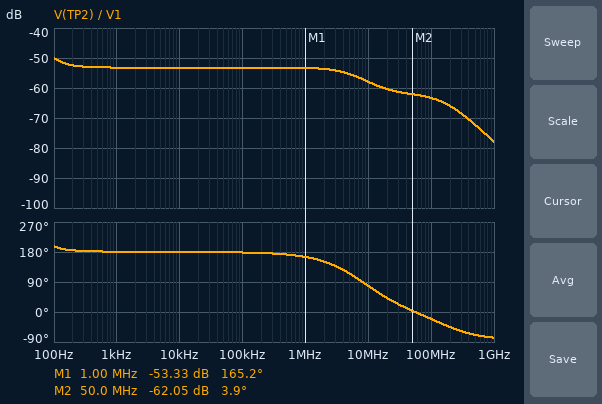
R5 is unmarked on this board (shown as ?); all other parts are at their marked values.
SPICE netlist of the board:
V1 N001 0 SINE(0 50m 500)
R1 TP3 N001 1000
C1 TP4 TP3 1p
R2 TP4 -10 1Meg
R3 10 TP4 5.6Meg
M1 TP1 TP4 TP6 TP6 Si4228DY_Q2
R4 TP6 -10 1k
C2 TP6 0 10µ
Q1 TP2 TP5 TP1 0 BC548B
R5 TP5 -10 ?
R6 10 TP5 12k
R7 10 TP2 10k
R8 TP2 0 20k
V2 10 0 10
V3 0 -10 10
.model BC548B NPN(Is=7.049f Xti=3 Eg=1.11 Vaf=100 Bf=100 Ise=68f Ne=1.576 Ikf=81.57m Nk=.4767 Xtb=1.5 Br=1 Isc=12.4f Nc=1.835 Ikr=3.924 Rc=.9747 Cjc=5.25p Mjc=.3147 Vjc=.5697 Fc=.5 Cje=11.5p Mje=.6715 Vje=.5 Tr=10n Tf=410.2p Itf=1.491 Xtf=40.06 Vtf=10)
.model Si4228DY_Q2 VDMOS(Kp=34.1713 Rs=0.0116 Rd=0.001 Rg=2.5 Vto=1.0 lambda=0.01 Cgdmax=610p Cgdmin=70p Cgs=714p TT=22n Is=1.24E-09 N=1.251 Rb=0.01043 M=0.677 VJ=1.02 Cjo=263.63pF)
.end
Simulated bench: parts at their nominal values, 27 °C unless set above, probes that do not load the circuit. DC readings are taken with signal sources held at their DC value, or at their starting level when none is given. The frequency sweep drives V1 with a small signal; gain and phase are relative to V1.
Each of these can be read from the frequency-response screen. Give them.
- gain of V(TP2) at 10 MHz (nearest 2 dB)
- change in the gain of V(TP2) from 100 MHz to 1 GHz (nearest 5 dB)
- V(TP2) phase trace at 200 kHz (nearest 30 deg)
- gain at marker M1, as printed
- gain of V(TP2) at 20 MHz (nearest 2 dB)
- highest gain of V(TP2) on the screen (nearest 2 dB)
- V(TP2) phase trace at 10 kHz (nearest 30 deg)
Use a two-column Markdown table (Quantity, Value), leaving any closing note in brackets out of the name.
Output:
| Quantity | Value |
|---|---|
| gain of V(TP2) at 10 MHz | -58 dB |
| change in the gain of V(TP2) from 100 MHz to 1 GHz | -15 dB |
| V(TP2) phase trace at 200 kHz | 180 deg |
| gain at marker M1, as printed | -53.33 dB |
| gain of V(TP2) at 20 MHz | -60 dB |
| highest gain of V(TP2) on the screen | -50 dB |
| V(TP2) phase trace at 10 kHz | 180 deg |
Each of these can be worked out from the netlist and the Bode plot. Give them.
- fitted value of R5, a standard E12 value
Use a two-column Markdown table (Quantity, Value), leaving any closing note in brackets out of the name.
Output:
| Quantity | Value |
|---|---|
| fitted value of R5, a standard E12 value | 2.7 kΩ |
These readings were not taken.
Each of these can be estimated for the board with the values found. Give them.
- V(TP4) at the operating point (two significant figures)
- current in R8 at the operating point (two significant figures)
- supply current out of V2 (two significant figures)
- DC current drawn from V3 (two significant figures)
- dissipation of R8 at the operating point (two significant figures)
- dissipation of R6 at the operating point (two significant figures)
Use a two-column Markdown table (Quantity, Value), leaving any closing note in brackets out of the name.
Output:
| Quantity | Value |
|---|---|
| V(TP4) at the operating point | -7.0 V |
| current in R8 at the operating point | 360 µA |
| supply current out of V2 | 3.1 mA |
| DC current drawn from V3 | 3.5 mA |
| dissipation of R8 at the operating point | 2.6 mW |
| dissipation of R6 at the operating point | 23 mW |
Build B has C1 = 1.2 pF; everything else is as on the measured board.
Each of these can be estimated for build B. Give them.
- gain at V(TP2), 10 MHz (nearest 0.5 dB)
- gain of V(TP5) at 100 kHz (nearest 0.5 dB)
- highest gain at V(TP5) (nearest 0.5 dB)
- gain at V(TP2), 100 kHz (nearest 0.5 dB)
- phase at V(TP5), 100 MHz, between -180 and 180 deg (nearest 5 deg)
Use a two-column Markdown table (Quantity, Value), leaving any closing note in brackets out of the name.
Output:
| Quantity | Value |
|---|---|
| gain at V(TP2), 10 MHz | -56.5 dB |
| gain of V(TP5) at 100 kHz | -52.5 dB |
| highest gain at V(TP5) | -46.0 dB |
| gain at V(TP2), 100 kHz | -51.5 dB |
| phase at V(TP5), 100 MHz, between -180 and 180 deg | -25 deg |
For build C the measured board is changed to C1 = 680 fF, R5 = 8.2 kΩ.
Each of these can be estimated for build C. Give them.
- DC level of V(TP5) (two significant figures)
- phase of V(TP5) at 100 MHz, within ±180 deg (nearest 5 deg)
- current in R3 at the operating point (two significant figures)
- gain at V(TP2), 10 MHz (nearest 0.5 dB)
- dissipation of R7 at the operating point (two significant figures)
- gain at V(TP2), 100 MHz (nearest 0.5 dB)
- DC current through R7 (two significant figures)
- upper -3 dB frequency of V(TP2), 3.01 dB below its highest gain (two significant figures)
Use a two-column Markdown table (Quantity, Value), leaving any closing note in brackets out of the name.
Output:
| Quantity | Value |
|---|---|
| DC level of V(TP5) | -4.3 V |
| phase of V(TP5) at 100 MHz, within ±180 deg | 0 deg |
| current in R3 at the operating point | 3.0 µA |
| gain at V(TP2), 10 MHz | -54.5 dB |
| dissipation of R7 at the operating point | 22 mW |
| gain at V(TP2), 100 MHz | -65.5 dB |
| DC current through R7 | 1.5 mA |
| upper -3 dB frequency of V(TP2), 3.01 dB below its highest gain | 110 Hz |
